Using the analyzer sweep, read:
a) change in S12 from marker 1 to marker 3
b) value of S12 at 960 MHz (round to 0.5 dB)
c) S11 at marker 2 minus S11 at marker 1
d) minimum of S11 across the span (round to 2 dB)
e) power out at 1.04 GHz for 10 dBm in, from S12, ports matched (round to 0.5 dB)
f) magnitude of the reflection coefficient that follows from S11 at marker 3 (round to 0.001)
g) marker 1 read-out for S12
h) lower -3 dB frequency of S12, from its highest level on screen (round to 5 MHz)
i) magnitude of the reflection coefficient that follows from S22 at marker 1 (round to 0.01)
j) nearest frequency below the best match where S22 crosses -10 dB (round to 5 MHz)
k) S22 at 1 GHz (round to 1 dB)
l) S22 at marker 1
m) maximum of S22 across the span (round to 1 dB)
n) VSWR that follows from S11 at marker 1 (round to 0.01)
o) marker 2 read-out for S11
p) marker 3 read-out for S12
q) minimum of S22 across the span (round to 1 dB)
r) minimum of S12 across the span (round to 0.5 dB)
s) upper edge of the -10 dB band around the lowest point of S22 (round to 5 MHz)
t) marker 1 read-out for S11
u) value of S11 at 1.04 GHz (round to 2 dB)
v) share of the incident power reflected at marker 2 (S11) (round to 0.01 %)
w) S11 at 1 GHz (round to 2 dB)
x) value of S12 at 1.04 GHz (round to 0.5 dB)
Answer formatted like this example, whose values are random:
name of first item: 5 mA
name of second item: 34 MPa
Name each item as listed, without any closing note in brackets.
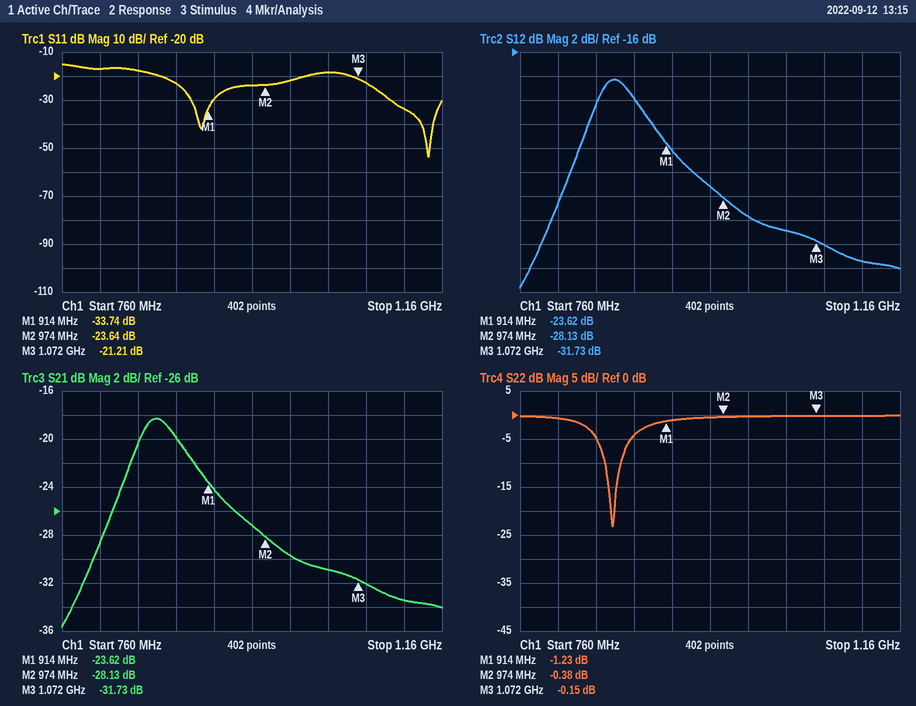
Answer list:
change in S12 from marker 1 to marker 3: -8.11 dB
value of S12 at 960 MHz: -27.0 dB
S11 at marker 2 minus S11 at marker 1: 10.10 dB
minimum of S11 across the span: -54 dB
power out at 1.04 GHz for 10 dBm in, from S12, ports matched: -21.0 dBm
magnitude of the reflection coefficient that follows from S11 at marker 3: 0.087
marker 1 read-out for S12: -23.62 dB
lower -3 dB frequency of S12, from its highest level on screen: 835 MHz
magnitude of the reflection coefficient that follows from S22 at marker 1: 0.87
nearest frequency below the best match where S22 crosses -10 dB: 850 MHz
S22 at 1 GHz: 0 dB
S22 at marker 1: -1.23 dB
maximum of S22 across the span: 0 dB
VSWR that follows from S11 at marker 1: 1.04
marker 2 read-out for S11: -23.64 dB
marker 3 read-out for S12: -31.73 dB
minimum of S22 across the span: -23 dB
minimum of S12 across the span: -35.5 dB
upper edge of the -10 dB band around the lowest point of S22: 865 MHz
marker 1 read-out for S11: -33.74 dB
value of S11 at 1.04 GHz: -18 dB
share of the incident power reflected at marker 2 (S11): 0.43 %
S11 at 1 GHz: -22 dB
value of S12 at 1.04 GHz: -31.0 dB
